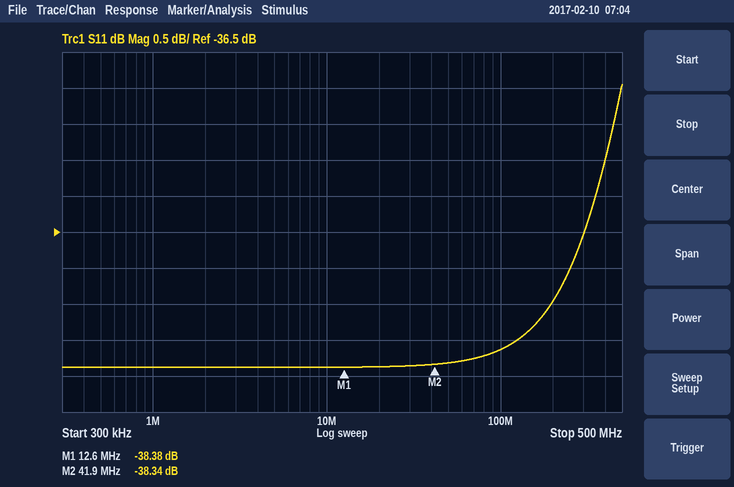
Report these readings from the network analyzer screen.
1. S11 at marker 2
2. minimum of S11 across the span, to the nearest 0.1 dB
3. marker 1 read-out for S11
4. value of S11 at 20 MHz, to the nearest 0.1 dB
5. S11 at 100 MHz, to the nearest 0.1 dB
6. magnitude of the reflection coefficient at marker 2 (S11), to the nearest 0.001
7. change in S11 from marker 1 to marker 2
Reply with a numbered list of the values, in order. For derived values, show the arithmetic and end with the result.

1. -38.34 dB
2. -38.4 dB
3. -38.38 dB
4. -38.4 dB
5. -38.1 dB
6. 10^(-38.34/20) ≈ 0.012
7. -38.34 − (-38.38) = 0.04 dB
